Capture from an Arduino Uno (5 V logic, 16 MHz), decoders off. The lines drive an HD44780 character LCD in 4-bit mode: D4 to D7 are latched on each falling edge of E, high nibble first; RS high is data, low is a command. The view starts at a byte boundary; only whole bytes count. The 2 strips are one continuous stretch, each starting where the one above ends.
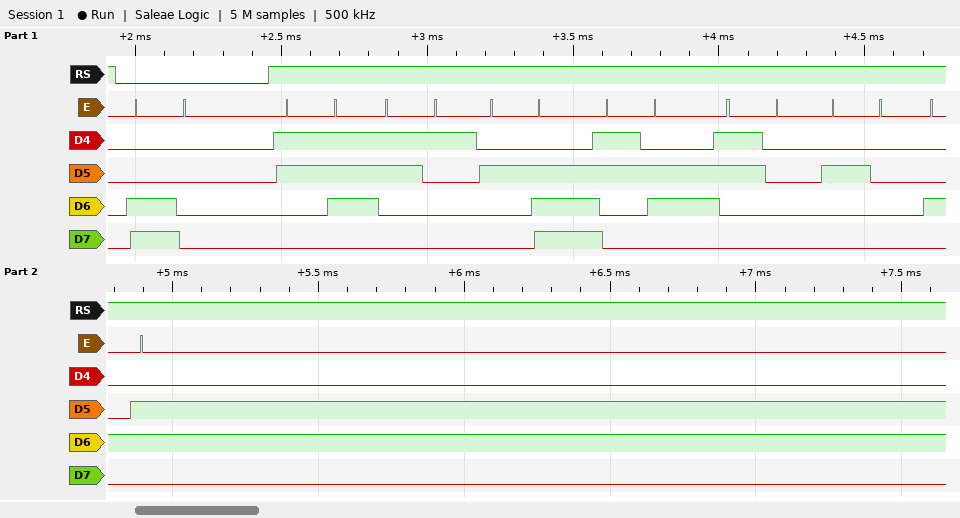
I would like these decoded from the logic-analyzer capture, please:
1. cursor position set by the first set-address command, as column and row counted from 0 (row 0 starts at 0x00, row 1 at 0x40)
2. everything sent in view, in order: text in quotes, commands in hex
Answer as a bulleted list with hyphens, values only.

- column 0, row 1
- 0xC0 "71.60 F"
